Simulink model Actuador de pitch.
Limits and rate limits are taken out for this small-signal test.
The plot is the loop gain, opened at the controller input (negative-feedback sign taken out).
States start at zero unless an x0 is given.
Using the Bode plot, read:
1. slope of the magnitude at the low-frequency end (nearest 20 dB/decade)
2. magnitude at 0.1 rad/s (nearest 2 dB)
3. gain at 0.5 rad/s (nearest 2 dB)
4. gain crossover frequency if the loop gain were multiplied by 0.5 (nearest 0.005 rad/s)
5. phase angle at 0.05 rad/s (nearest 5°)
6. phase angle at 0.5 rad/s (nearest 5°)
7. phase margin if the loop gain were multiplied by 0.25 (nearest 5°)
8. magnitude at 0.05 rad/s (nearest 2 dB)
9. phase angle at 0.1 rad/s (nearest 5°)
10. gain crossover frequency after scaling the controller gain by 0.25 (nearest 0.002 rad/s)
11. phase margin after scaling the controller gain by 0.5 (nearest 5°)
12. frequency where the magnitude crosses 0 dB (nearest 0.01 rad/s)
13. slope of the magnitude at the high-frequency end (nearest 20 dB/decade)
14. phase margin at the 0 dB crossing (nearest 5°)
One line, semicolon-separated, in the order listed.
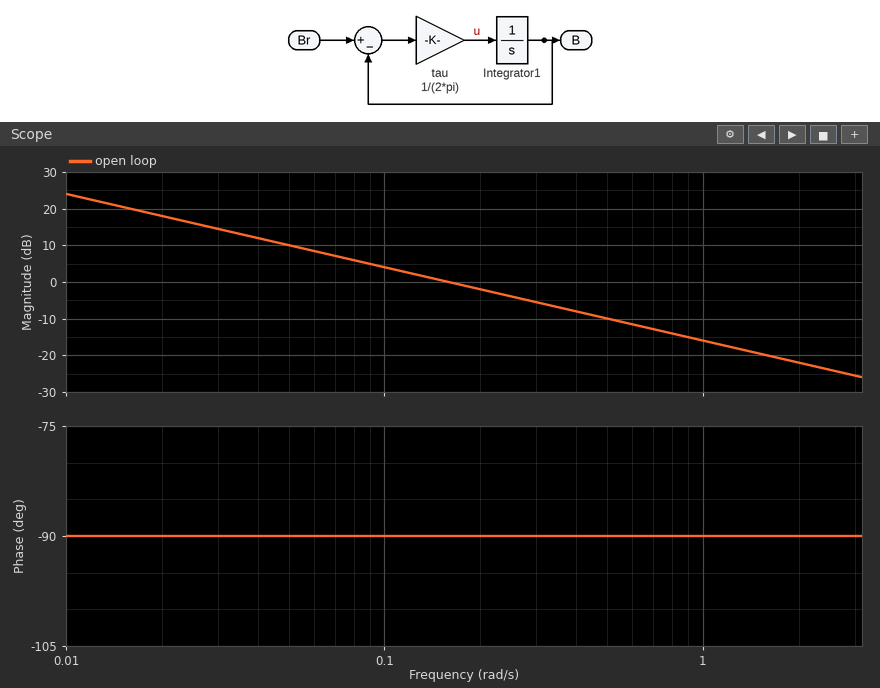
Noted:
-20 dB/decade; 4 dB; -10 dB; 0.080 rad/s; -90°; -90°; 90°; 10 dB; -90°; 0.040 rad/s; 90°; 0.16 rad/s; -20 dB/decade; 90°
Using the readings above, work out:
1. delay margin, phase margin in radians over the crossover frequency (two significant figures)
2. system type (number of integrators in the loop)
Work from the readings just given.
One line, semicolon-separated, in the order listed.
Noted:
9.8 s; 1
